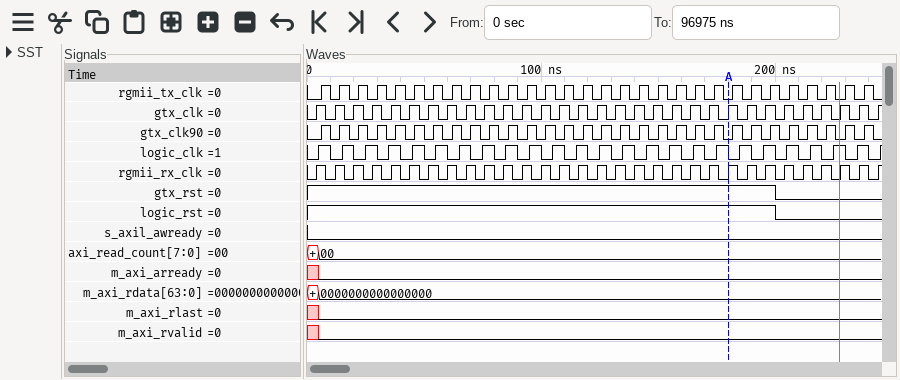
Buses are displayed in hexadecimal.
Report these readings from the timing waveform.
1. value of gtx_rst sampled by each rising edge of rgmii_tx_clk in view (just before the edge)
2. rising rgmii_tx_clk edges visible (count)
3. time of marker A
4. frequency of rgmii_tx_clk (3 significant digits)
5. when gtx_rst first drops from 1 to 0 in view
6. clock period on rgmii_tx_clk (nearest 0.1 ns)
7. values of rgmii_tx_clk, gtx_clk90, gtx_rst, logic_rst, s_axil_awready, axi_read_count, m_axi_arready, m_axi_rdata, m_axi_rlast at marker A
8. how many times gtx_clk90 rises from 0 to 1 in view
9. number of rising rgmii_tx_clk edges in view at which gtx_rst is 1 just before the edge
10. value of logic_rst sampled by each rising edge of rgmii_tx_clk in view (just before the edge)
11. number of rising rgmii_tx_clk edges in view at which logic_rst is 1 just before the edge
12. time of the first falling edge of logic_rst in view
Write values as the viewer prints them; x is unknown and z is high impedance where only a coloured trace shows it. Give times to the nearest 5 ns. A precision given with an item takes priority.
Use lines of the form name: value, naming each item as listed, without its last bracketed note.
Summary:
value of gtx_rst sampled by each rising edge of rgmii_tx_clk in view: 1 1 1 1 1 1 1 1 1 1 1 1 1 1 1 1 1 1 1 1 1 1 1 1 1 0 0 0 0 0
rising rgmii_tx_clk edges visible: 30
time of marker A: 180 ns
frequency of rgmii_tx_clk: 125 MHz
when gtx_rst first drops from 1 to 0 in view: 200 ns
clock period on rgmii_tx_clk: 8 ns
values of rgmii_tx_clk, gtx_clk90, gtx_rst, logic_rst, s_axil_awready, axi_read_count, m_axi_arready, m_axi_rdata, m_axi_rlast at marker A: rgmii_tx_clk=0, gtx_clk90=0, gtx_rst=1, logic_rst=1, s_axil_awready=0, axi_read_count=00, m_axi_arready=0, m_axi_rdata=0000000000000000, m_axi_rlast=0
how many times gtx_clk90 rises from 0 to 1 in view: 30
number of rising rgmii_tx_clk edges in view at which gtx_rst is 1 just before the edge: 25
value of logic_rst sampled by each rising edge of rgmii_tx_clk in view: 1 1 1 1 1 1 1 1 1 1 1 1 1 1 1 1 1 1 1 1 1 1 1 1 1 0 0 0 0 0
number of rising rgmii_tx_clk edges in view at which logic_rst is 1 just before the edge: 25
time of the first falling edge of logic_rst in view: 200 ns
